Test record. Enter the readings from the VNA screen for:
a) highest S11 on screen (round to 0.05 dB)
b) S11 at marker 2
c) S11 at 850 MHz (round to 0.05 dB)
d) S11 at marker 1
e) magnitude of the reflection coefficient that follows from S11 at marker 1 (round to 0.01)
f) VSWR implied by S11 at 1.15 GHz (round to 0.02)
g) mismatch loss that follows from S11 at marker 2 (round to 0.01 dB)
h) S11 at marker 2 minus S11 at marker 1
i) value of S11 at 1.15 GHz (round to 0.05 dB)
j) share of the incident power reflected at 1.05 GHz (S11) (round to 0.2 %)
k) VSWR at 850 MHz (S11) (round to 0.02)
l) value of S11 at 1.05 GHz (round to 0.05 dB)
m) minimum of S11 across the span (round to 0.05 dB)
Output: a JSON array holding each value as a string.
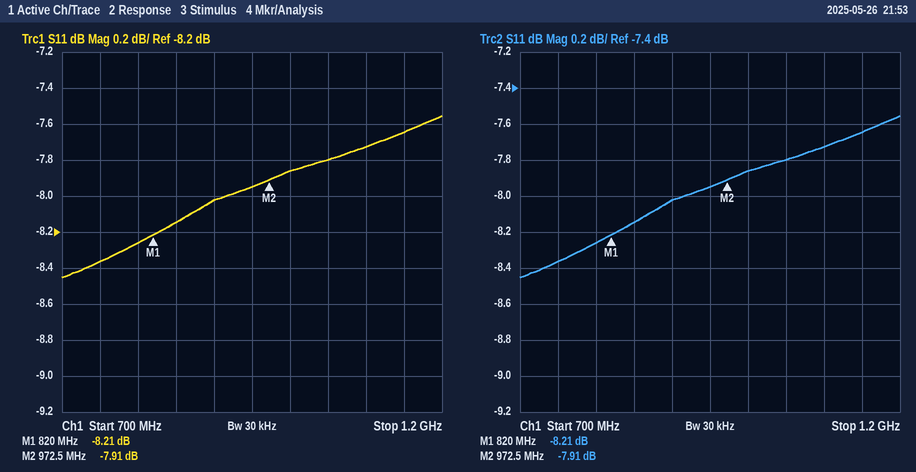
["-7.55 dB", "-7.91 dB", "-8.15 dB", "-8.21 dB", "0.39", "2.42", "0.77 dB", "0.30 dB", "-7.65 dB", "16.6 %", "2.28", "-7.80 dB", "-8.45 dB"]
